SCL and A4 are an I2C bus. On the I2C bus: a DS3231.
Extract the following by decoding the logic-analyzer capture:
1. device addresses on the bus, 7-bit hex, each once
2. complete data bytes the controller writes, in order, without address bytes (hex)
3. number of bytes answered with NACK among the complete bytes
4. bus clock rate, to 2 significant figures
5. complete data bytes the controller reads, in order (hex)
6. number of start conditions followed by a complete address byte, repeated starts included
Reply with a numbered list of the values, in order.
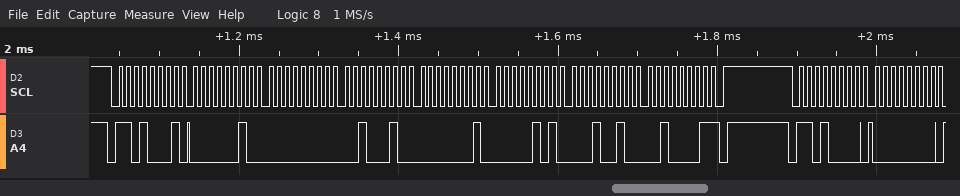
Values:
1. 0x68
2. 00
3. 1
4. 100 kHz
5. 02 00 22 01 05 12 21
6. 2
